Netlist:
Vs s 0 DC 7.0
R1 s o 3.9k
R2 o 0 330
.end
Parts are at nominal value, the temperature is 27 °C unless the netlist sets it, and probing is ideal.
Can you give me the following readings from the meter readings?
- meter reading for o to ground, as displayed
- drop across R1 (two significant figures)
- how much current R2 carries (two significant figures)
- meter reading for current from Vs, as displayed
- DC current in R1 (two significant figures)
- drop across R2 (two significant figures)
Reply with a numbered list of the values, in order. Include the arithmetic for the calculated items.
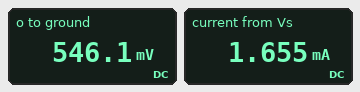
1. 546.1 mV
2. 7 V - 546.1 mV = 6.5 V
3. (546.1 mV) / 330 Ω = 1.7 mA
4. 1.655 mA
5. (7 V - 546.1 mV) / 3.9 kΩ = 1.7 mA
6. 546.1 mV = 550 mV
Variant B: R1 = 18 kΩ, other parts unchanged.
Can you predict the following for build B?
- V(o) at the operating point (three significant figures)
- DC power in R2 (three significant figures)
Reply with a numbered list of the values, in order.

1. 126 mV
2. 48.1 µW
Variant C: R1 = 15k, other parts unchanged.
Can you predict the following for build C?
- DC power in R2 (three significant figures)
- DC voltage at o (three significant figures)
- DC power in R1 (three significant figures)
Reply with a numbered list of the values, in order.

1. 68.8 µW
2. 151 mV
3. 3.13 mW
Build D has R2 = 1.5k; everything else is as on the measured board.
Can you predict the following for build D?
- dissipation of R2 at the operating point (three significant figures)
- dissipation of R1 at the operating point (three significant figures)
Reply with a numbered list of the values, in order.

1. 2.52 mW
2. 6.55 mW
